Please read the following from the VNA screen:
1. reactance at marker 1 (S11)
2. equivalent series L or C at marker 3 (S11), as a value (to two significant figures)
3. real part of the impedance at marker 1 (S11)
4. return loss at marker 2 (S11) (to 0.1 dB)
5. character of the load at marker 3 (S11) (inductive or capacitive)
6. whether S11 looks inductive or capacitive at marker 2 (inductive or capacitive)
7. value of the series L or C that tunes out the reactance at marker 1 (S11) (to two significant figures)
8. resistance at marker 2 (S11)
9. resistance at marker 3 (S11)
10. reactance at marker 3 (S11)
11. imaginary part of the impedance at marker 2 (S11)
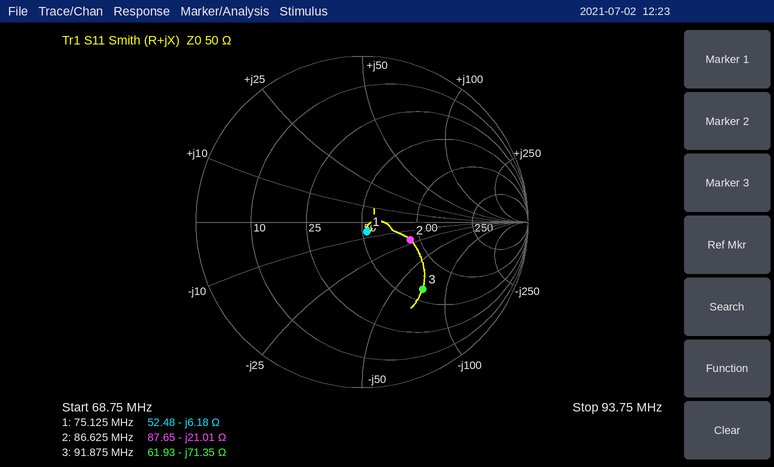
-6.18 Ω
24 pF
52.48 Ω
10.2 dB
capacitive
capacitive
13 nH
87.65 Ω
61.93 Ω
-71.35 Ω
-21.01 Ω
